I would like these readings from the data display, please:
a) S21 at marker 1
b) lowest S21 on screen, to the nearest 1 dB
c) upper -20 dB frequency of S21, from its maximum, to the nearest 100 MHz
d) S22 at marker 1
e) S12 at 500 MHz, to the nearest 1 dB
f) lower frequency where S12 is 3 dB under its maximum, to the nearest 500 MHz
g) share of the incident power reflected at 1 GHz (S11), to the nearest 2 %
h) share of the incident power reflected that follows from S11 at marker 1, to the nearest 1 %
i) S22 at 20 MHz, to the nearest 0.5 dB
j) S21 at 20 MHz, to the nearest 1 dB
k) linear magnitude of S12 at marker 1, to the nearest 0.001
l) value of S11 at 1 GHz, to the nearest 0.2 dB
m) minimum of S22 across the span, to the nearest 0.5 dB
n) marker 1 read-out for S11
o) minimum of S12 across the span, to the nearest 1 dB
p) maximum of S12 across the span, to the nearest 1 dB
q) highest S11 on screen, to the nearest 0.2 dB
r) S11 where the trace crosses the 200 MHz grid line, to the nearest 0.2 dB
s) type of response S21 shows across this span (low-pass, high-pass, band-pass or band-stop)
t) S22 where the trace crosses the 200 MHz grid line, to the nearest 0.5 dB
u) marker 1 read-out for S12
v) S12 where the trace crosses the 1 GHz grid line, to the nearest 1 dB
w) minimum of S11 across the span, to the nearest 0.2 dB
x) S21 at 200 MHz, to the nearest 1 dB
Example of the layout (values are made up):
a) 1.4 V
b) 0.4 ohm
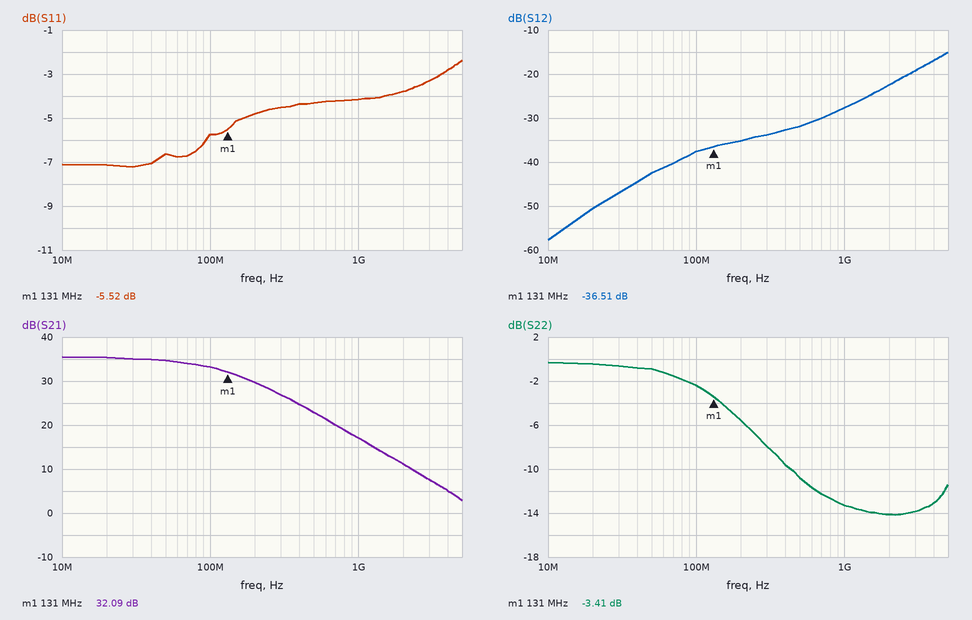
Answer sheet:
a) 32.09 dB
b) 3 dB
c) 1.2 GHz
d) -3.41 dB
e) -32 dB
f) 3.5 GHz
g) 38 %
h) 28 %
i) -0.5 dB
j) 35 dB
k) 0.015
l) -4.2 dB
m) -14.0 dB
n) -5.52 dB
o) -58 dB
p) -15 dB
q) -2.4 dB
r) -4.8 dB
s) low-pass
t) -5.5 dB
u) -36.51 dB
v) -28 dB
w) -7.2 dB
x) 30 dB
